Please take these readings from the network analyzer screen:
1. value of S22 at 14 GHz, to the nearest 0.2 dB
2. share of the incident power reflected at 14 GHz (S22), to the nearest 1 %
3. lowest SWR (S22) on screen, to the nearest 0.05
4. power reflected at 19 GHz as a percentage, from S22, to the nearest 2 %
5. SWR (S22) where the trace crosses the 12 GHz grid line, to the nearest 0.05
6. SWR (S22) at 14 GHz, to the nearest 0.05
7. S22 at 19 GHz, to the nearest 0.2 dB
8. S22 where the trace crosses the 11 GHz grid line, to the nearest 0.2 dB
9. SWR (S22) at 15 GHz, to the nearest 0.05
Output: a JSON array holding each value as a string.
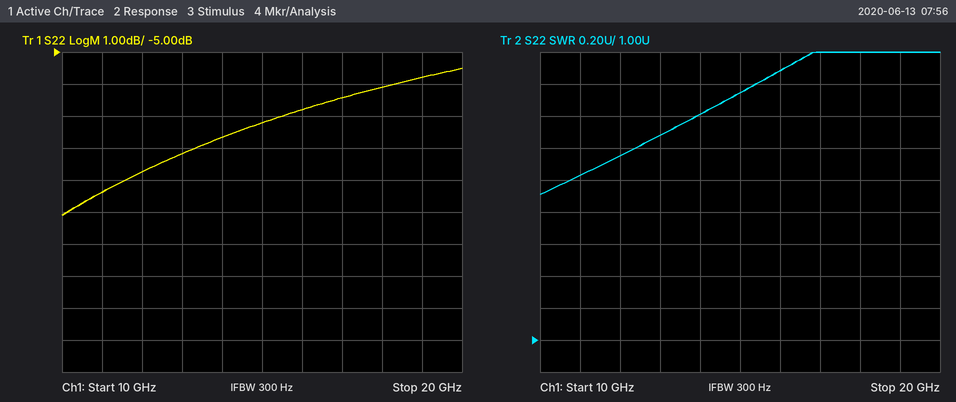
["-7.6 dB", "17 %", "1.90", "26 %", "2.15", "2.40", "-5.8 dB", "-9.4 dB", "2.55"]
